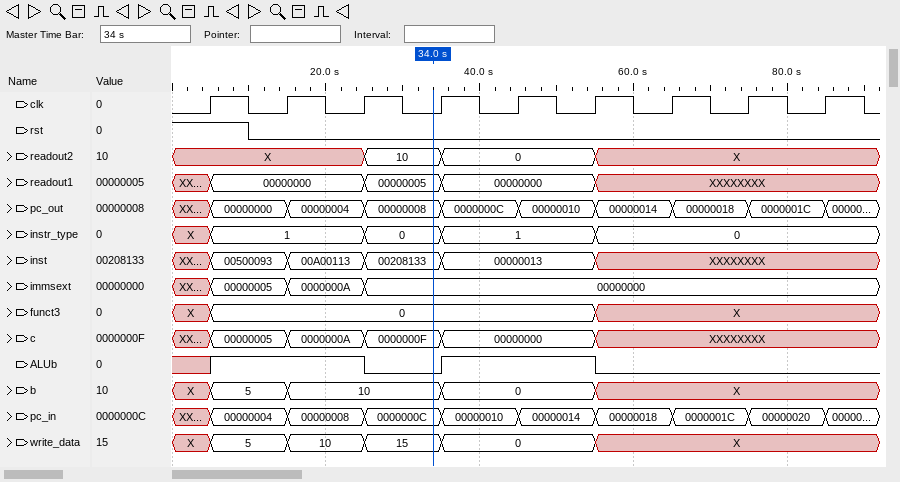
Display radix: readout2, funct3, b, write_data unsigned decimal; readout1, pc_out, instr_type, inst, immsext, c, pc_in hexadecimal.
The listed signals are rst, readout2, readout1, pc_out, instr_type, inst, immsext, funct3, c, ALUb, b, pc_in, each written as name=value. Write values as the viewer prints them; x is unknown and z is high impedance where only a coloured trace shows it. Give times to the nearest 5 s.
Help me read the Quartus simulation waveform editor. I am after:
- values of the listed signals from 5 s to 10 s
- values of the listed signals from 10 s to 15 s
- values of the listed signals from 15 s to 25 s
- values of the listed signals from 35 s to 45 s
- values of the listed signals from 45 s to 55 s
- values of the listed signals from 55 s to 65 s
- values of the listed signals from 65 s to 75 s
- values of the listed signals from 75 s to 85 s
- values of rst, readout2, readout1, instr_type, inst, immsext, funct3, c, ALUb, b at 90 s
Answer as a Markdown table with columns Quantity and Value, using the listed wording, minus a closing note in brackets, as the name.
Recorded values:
| Quantity | Value |
|---|---|
| values of the listed signals from 5 s to 10 s | rst=1, readout2=X, readout1=00000000, pc_out=00000000, instr_type=1, inst=00500093, immsext=00000005, funct3=0, c=00000005, ALUb=1, b=5, pc_in=00000004 |
| values of the listed signals from 10 s to 15 s | rst=0, readout2=X, readout1=00000000, pc_out=00000000, instr_type=1, inst=00500093, immsext=00000005, funct3=0, c=00000005, ALUb=1, b=5, pc_in=00000004 |
| values of the listed signals from 15 s to 25 s | rst=0, readout2=X, readout1=00000000, pc_out=00000004, instr_type=1, inst=00A00113, immsext=0000000A, funct3=0, c=0000000A, ALUb=1, b=10, pc_in=00000008 |
| values of the listed signals from 35 s to 45 s | rst=0, readout2=0, readout1=00000000, pc_out=0000000C, instr_type=1, inst=00000013, immsext=00000000, funct3=0, c=00000000, ALUb=1, b=0, pc_in=00000010 |
| values of the listed signals from 45 s to 55 s | rst=0, readout2=0, readout1=00000000, pc_out=00000010, instr_type=1, inst=00000013, immsext=00000000, funct3=0, c=00000000, ALUb=1, b=0, pc_in=00000014 |
| values of the listed signals from 55 s to 65 s | rst=0, readout2=X, readout1=XXXXXXXX, pc_out=00000014, instr_type=0, inst=XXXXXXXX, immsext=00000000, funct3=X, c=XXXXXXXX, ALUb=0, b=X, pc_in=00000018 |
| values of the listed signals from 65 s to 75 s | rst=0, readout2=X, readout1=XXXXXXXX, pc_out=00000018, instr_type=0, inst=XXXXXXXX, immsext=00000000, funct3=X, c=XXXXXXXX, ALUb=0, b=X, pc_in=0000001C |
| values of the listed signals from 75 s to 85 s | rst=0, readout2=X, readout1=XXXXXXXX, pc_out=0000001C, instr_type=0, inst=XXXXXXXX, immsext=00000000, funct3=X, c=XXXXXXXX, ALUb=0, b=X, pc_in=00000020 |
| values of rst, readout2, readout1, instr_type, inst, immsext, funct3, c, ALUb, b at 90 s | rst=0, readout2=X, readout1=XXXXXXXX, instr_type=0, inst=XXXXXXXX, immsext=00000000, funct3=X, c=XXXXXXXX, ALUb=0, b=X |
